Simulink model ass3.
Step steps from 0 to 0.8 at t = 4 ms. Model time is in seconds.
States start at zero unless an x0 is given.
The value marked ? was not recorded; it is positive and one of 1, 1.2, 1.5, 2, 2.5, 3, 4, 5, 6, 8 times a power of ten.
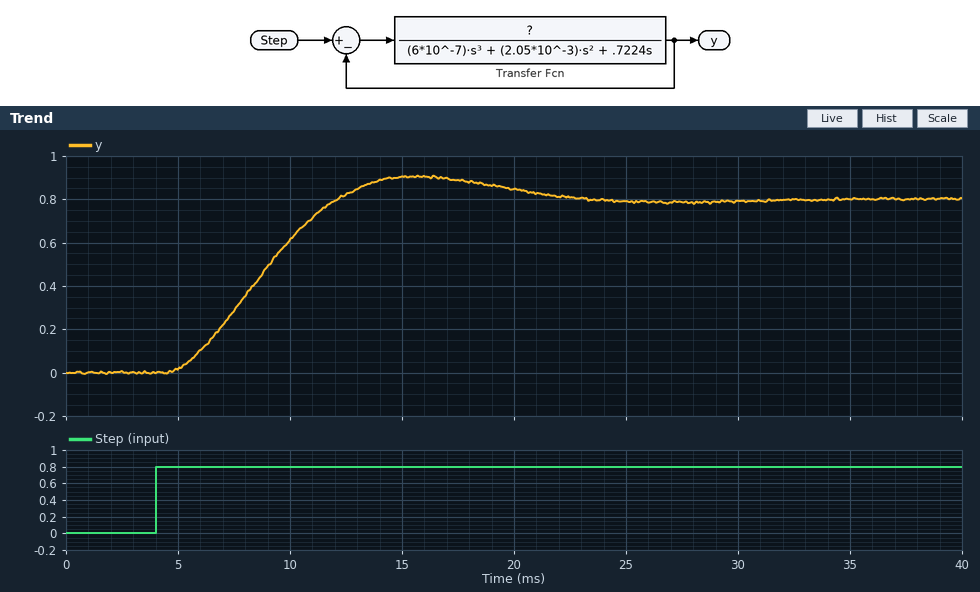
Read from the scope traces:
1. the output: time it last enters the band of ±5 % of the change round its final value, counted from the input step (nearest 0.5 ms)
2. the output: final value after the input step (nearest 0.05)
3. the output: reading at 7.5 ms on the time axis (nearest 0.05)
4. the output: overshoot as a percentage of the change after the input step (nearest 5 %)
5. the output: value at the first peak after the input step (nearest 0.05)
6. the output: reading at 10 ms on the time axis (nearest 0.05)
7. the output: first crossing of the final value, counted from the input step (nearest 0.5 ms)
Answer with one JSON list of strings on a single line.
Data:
["16.5 ms", "0.80", "0.30", "15 %", "0.90", "0.60", "8.0 ms"]
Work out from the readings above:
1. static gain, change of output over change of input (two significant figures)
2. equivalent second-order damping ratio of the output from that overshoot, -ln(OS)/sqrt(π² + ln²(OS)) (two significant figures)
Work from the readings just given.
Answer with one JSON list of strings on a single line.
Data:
["1.0", "0.52"]
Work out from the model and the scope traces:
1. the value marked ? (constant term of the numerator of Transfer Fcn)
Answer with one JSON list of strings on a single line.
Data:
["200"]
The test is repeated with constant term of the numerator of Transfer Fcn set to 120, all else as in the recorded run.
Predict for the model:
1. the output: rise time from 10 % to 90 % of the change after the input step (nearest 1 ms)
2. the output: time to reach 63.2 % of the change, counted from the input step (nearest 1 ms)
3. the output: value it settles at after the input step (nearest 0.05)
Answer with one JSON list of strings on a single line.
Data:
["9 ms", "7 ms", "0.80"]
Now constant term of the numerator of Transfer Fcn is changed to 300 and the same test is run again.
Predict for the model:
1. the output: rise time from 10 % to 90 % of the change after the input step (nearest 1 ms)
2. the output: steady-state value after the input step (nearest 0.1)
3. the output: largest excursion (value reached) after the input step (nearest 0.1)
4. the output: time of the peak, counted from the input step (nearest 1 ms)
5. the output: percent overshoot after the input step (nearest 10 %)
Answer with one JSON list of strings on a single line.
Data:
["4 ms", "0.8", "1.0", "9 ms", "20 %"]
